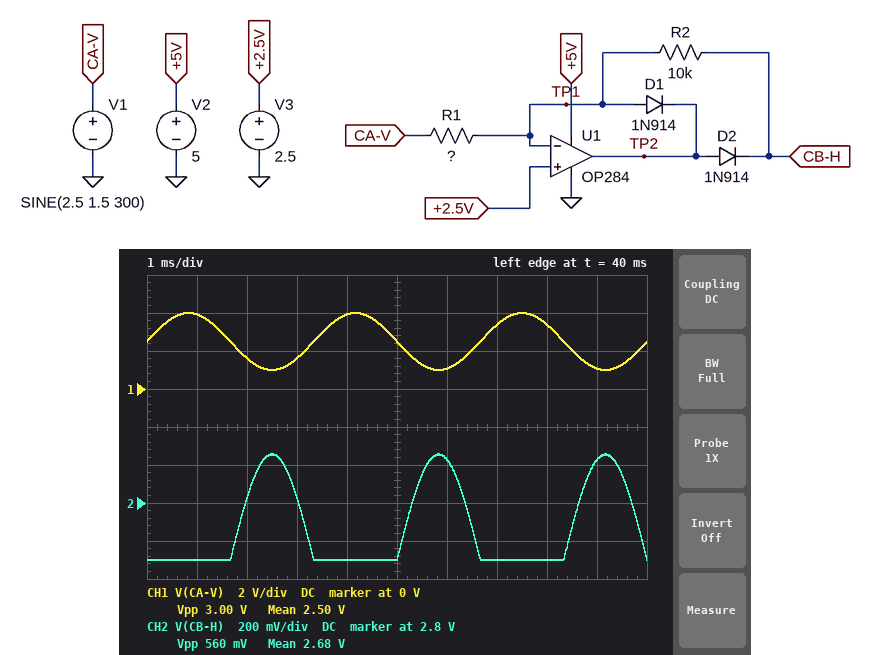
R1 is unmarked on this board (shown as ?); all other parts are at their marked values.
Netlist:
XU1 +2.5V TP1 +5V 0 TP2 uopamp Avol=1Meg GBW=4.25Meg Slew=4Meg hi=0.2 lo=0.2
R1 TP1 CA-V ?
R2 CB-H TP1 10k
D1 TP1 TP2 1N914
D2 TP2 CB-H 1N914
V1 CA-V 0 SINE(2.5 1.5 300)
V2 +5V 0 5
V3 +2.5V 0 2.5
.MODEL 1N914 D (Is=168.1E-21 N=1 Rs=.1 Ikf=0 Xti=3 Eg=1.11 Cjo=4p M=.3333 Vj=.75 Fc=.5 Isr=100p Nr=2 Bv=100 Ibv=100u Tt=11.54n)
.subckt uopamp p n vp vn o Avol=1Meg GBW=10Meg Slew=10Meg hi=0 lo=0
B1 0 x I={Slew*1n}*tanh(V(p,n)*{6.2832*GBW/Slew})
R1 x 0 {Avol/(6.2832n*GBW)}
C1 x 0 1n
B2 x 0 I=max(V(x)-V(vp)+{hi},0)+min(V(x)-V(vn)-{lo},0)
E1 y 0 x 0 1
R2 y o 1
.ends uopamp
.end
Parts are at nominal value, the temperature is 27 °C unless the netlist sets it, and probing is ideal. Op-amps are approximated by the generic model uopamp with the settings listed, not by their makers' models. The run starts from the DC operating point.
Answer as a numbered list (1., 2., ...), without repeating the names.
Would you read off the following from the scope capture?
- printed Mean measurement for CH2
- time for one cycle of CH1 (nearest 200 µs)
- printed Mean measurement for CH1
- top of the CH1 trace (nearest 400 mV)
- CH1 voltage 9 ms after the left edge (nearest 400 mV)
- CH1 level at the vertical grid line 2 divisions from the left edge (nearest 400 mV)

1. 2.68 V
2. 3.4 ms
3. 2.50 V
4. 4.0 V
5. 1.2 V
6. 1.6 V
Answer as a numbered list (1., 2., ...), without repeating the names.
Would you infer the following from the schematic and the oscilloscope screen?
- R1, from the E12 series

1. 27 kΩ
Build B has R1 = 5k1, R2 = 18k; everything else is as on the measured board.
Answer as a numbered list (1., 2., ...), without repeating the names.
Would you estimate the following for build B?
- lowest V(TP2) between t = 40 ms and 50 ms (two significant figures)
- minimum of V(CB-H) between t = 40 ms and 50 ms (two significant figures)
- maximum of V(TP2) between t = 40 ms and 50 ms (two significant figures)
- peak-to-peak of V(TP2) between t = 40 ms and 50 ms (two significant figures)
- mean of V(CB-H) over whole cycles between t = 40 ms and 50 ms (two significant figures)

1. 1.7 V
2. 2.5 V
3. 4.8 V
4. 3.1 V
5. 3.2 V
